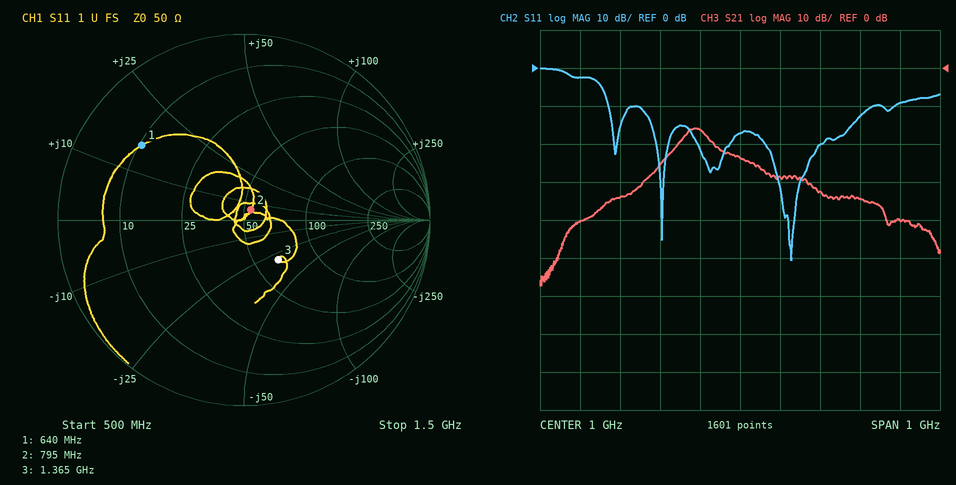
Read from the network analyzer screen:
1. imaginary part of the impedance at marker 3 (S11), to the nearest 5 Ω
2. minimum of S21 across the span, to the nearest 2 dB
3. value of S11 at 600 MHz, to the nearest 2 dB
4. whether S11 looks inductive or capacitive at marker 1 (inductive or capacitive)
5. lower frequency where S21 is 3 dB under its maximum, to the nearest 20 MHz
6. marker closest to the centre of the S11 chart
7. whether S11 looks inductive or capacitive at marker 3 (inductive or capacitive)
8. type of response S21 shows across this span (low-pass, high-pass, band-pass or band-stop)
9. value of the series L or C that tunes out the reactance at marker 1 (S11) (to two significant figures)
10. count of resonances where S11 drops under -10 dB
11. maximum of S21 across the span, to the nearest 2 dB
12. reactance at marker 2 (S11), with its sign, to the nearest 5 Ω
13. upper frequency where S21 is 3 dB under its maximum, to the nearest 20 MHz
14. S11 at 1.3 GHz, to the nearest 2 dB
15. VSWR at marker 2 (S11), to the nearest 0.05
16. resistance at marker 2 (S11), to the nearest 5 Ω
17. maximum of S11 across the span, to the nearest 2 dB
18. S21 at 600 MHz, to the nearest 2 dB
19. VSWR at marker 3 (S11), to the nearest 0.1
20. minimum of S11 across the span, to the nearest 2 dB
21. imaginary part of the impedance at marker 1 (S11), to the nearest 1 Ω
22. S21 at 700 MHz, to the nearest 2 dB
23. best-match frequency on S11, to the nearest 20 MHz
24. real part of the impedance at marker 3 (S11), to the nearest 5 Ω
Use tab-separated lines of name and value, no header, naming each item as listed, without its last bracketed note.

imaginary part of the impedance at marker 3 (S11), to the nearest 5 Ω	-30 Ω
minimum of S21 across the span, to the nearest 2 dB	-58 dB
value of S11 at 600 MHz, to the nearest 2 dB	-2 dB
whether S11 looks inductive or capacitive at marker 1	inductive
lower frequency where S21 is 3 dB under its maximum, to the nearest 20 MHz	860 MHz
marker closest to the centre of the S11 chart	marker 2
whether S11 looks inductive or capacitive at marker 3	capacitive
type of response S21 shows across this span	band-pass
value of the series L or C that tunes out the reactance at marker 1 (S11)	16 pF
count of resonances where S11 drops under -10 dB	4
maximum of S21 across the span, to the nearest 2 dB	-16 dB
reactance at marker 2 (S11), with its sign, to the nearest 5 Ω	+5 Ω
upper frequency where S21 is 3 dB under its maximum, to the nearest 20 MHz	920 MHz
S11 at 1.3 GHz, to the nearest 2 dB	-12 dB
VSWR at marker 2 (S11), to the nearest 0.05	1.15
resistance at marker 2 (S11), to the nearest 5 Ω	55 Ω
maximum of S11 across the span, to the nearest 2 dB	0 dB
S21 at 600 MHz, to the nearest 2 dB	-40 dB
VSWR at marker 3 (S11), to the nearest 0.1	1.8
minimum of S11 across the span, to the nearest 2 dB	-50 dB
imaginary part of the impedance at marker 1 (S11), to the nearest 1 Ω	+16 Ω
S21 at 700 MHz, to the nearest 2 dB	-34 dB
best-match frequency on S11, to the nearest 20 MHz	1.12 GHz
real part of the impedance at marker 3 (S11), to the nearest 5 Ω	65 Ω
